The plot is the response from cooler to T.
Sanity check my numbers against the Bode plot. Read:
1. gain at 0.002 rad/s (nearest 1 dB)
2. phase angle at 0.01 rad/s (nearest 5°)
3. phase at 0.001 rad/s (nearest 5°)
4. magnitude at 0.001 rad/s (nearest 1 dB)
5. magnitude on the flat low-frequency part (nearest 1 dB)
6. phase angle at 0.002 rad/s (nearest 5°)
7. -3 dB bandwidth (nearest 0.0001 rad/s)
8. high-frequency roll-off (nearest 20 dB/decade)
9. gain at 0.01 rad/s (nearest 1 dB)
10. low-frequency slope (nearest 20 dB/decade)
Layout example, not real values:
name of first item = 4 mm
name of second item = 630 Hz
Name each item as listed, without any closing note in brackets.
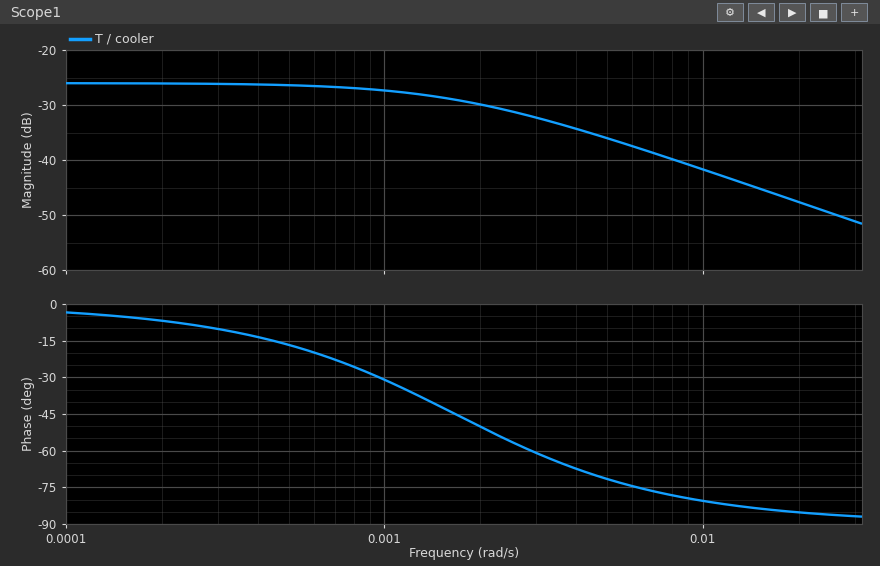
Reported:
gain at 0.002 rad/s = -30 dB
phase angle at 0.01 rad/s = -80°
phase at 0.001 rad/s = -30°
magnitude at 0.001 rad/s = -27 dB
magnitude on the flat low-frequency part = -26 dB
phase angle at 0.002 rad/s = -50°
-3 dB bandwidth = 0.0017 rad/s
high-frequency roll-off = -20 dB/decade
gain at 0.01 rad/s = -42 dB
low-frequency slope = 0 dB/decade
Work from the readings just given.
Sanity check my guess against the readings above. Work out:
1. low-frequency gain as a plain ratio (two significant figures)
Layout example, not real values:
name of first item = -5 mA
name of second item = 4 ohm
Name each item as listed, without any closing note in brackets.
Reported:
low-frequency gain as a plain ratio = 0.050
